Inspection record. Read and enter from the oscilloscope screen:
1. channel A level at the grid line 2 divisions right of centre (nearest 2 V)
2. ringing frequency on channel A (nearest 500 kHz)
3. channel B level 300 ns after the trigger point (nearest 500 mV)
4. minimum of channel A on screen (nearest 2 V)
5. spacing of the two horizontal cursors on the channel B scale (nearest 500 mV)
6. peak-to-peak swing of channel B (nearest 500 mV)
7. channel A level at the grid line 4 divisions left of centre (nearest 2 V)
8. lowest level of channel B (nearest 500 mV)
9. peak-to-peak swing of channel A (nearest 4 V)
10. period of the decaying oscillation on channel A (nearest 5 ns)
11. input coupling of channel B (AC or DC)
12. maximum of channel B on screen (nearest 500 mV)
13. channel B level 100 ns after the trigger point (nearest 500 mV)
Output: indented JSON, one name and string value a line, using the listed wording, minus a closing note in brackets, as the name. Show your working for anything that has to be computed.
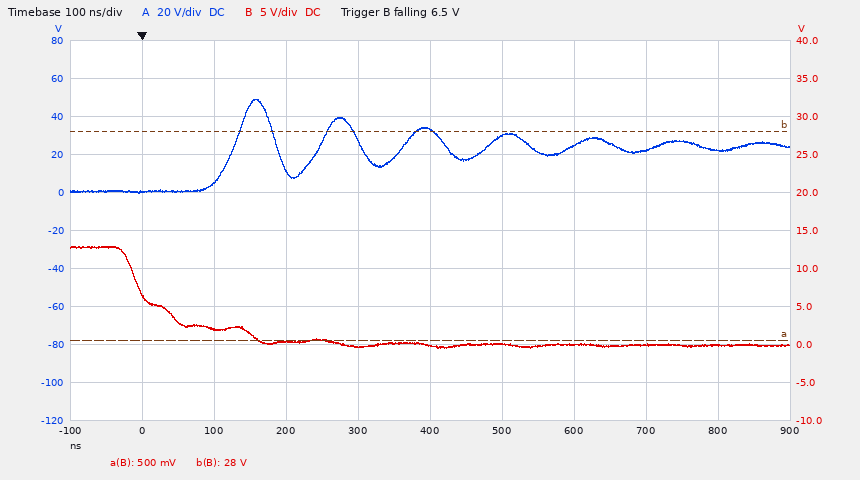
{
  "channel A level at the grid line 2 divisions right of centre": "24 V",
  "ringing frequency on channel A": "1 / 115 ns ≈ 8.70 MHz, so 8.5 MHz to the nearest 500 kHz",
  "channel B level 300 ns after the trigger point": "-500 mV",
  "minimum of channel A on screen": "0 V",
  "spacing of the two horizontal cursors on the channel B scale": "27.5 V",
  "peak-to-peak swing of channel B": "13.0 V − (-500 mV) = 13.5 V",
  "channel A level at the grid line 4 divisions left of centre": "0 V",
  "lowest level of channel B": "-500 mV",
  "peak-to-peak swing of channel A": "48 V",
  "period of the decaying oscillation on channel A": "115 ns",
  "input coupling of channel B": "DC",
  "maximum of channel B on screen": "13.0 V",
  "channel B level 100 ns after the trigger point": "2.0 V"
}
